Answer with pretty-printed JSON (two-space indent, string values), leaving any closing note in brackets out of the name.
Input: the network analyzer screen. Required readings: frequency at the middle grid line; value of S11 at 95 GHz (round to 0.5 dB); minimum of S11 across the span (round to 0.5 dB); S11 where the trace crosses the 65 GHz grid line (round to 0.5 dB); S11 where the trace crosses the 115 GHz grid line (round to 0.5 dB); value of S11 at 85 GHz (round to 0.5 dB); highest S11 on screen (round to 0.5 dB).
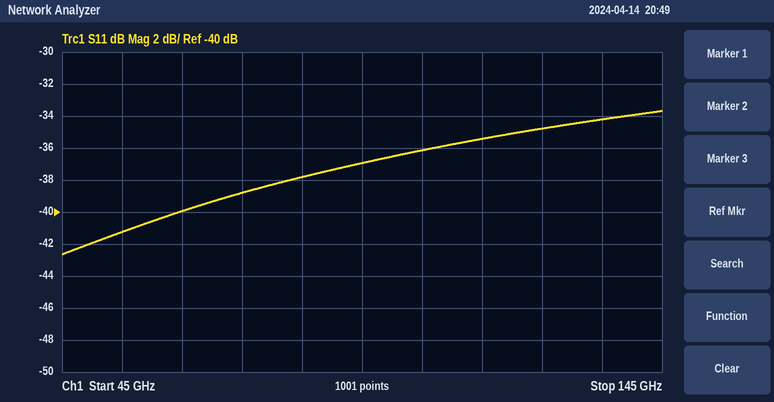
{
  "frequency at the middle grid line": "95 GHz",
  "value of S11 at 95 GHz": "-37.0 dB",
  "minimum of S11 across the span": "-42.5 dB",
  "S11 where the trace crosses the 65 GHz grid line": "-40.0 dB",
  "S11 where the trace crosses the 115 GHz grid line": "-35.5 dB",
  "value of S11 at 85 GHz": "-38.0 dB",
  "highest S11 on screen": "-33.5 dB"
}
